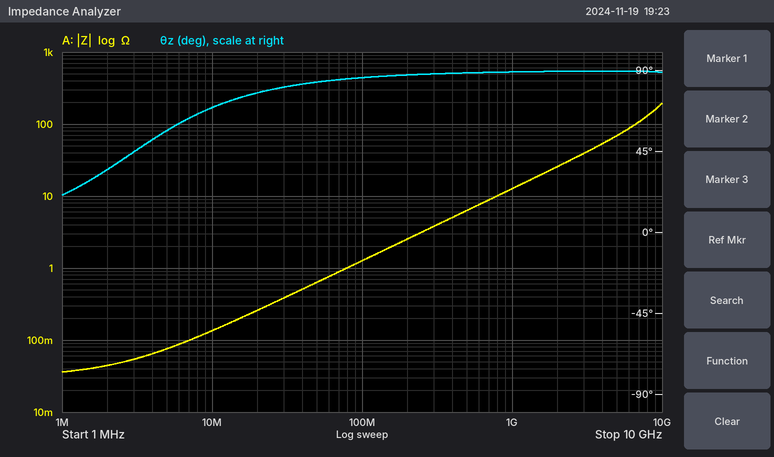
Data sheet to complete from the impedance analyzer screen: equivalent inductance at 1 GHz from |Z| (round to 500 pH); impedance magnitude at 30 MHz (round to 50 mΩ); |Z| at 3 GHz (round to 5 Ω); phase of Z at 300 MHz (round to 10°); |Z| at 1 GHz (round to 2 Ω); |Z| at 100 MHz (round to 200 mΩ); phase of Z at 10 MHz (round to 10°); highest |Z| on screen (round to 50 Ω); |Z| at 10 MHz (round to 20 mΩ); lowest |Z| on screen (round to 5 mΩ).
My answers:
2.0 nH
400 mΩ
40 Ω
90°
12 Ω
1.2 Ω
70°
200 Ω
140 mΩ
35 mΩ
